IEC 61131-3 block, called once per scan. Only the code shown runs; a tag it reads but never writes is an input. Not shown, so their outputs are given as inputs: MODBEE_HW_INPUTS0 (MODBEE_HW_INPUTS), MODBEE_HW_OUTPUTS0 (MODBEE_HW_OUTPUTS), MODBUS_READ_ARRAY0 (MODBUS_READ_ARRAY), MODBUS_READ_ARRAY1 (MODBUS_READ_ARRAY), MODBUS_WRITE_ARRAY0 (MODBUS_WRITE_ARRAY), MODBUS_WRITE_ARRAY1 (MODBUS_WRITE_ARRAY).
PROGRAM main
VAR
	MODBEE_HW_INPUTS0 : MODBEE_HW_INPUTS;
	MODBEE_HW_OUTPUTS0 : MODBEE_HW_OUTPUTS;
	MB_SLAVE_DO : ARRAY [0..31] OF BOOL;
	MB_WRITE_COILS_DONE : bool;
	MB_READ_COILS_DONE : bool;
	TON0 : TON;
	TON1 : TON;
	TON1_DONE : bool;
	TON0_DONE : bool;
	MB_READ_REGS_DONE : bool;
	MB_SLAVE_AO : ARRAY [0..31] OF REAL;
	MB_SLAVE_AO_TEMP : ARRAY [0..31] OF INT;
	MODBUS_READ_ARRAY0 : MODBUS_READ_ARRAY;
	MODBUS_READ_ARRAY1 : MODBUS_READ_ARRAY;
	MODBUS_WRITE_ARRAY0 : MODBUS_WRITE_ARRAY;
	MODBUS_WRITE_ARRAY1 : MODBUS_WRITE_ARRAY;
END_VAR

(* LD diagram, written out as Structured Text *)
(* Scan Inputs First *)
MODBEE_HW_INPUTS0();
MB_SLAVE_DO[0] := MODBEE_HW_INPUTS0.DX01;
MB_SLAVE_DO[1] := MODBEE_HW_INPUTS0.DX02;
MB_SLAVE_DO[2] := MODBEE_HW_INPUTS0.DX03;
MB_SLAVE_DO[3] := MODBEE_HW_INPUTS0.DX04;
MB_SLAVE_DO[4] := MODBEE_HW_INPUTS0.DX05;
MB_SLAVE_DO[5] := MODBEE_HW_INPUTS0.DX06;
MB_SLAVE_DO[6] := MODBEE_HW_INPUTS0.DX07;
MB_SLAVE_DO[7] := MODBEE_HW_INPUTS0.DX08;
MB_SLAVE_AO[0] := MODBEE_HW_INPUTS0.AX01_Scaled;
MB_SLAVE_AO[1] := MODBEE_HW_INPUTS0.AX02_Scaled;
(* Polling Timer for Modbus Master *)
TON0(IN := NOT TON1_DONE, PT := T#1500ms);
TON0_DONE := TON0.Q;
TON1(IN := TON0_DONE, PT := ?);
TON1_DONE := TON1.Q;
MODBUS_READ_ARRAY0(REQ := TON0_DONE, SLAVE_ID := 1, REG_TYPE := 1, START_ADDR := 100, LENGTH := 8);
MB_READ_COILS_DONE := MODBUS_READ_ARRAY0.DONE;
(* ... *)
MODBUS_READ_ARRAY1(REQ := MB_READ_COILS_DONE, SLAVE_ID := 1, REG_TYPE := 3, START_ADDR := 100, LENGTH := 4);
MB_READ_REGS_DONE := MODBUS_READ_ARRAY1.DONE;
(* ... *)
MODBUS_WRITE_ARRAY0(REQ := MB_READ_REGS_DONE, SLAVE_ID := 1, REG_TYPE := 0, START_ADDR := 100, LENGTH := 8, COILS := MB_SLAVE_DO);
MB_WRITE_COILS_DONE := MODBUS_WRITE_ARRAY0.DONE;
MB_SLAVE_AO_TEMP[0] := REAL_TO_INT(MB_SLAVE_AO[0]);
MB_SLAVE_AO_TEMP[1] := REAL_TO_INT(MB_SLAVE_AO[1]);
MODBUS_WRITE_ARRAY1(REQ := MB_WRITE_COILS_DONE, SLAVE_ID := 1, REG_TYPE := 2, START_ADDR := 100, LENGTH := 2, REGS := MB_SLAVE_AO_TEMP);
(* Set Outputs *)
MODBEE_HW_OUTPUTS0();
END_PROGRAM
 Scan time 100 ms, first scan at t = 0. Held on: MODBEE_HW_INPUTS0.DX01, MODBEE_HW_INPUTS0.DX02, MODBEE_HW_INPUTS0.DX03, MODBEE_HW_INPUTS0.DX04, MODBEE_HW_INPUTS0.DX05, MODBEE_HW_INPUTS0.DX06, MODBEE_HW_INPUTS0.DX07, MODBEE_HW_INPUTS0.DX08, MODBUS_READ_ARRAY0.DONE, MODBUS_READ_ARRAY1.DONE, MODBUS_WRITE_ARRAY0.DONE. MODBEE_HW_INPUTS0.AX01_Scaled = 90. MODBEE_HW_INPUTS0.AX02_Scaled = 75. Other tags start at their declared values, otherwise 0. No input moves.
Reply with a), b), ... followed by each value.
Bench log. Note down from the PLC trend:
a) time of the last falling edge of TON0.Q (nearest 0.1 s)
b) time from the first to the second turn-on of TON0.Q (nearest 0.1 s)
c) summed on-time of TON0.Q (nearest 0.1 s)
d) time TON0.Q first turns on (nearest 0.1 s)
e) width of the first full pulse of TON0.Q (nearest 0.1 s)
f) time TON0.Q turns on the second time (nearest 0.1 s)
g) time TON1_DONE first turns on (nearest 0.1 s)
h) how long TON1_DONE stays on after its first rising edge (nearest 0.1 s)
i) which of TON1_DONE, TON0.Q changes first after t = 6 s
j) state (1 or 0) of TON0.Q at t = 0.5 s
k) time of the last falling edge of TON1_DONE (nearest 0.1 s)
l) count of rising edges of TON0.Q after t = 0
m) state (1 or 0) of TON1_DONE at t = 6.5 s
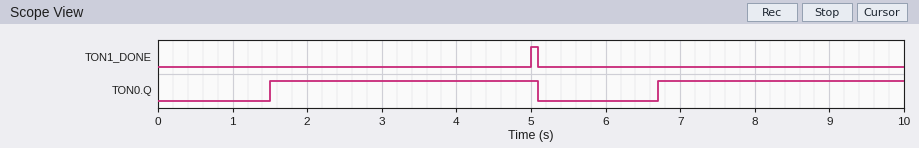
a) 5.1 s
b) 5.2 s
c) 6.9 s
d) 1.5 s
e) 3.6 s
f) 6.7 s
g) 5.0 s
h) 0.1 s
i) TON0.Q
j) 0
k) 5.1 s
l) 2
m) 0
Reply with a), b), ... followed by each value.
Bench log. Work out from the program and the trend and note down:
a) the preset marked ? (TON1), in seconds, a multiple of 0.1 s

a) 3.5 s
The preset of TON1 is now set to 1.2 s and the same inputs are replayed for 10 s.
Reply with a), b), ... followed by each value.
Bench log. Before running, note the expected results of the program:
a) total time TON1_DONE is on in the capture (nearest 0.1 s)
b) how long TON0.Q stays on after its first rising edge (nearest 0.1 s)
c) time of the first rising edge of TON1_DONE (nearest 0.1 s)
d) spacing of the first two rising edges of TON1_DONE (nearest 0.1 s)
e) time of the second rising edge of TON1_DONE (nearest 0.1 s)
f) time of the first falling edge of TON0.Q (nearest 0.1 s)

a) 0.3 s
b) 1.3 s
c) 2.7 s
d) 2.9 s
e) 5.6 s
f) 2.8 s
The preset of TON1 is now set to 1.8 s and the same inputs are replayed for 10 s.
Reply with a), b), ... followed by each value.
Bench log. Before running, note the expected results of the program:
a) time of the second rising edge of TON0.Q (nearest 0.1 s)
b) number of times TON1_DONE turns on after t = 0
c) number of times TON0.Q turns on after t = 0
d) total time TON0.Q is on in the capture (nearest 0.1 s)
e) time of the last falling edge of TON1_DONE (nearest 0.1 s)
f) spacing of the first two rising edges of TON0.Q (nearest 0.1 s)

a) 5.0 s
b) 2
c) 3
d) 5.3 s
e) 6.9 s
f) 3.5 s
